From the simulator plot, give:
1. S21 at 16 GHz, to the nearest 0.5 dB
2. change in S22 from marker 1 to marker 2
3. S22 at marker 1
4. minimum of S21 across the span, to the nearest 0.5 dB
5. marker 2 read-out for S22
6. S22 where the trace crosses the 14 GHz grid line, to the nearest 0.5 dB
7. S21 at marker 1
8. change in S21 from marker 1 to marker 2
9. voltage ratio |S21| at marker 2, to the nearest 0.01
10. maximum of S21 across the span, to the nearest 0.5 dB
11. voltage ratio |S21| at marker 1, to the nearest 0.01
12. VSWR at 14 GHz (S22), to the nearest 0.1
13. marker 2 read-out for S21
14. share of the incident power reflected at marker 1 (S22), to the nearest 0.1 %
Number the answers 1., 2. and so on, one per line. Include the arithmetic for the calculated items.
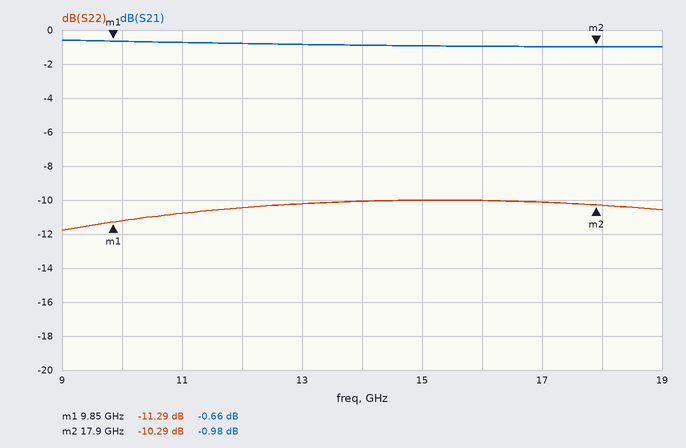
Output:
1. -1.0 dB
2. -10.29 − (-11.29) = 1.00 dB
3. -11.29 dB
4. -1.0 dB
5. -10.29 dB
6. -10.0 dB
7. -0.66 dB
8. -0.98 − (-0.66) = -0.32 dB
9. 10^(-0.98/20) ≈ 0.89
10. -0.5 dB
11. 10^(-0.66/20) ≈ 0.93
12. |Γ| = 10^(-10/20) = 0.3162; VSWR = (1 + 0.3162)/(1 − 0.3162) ≈ 1.9
13. -0.98 dB
14. 10^(-11.29/10) ≈ 7.4 %
